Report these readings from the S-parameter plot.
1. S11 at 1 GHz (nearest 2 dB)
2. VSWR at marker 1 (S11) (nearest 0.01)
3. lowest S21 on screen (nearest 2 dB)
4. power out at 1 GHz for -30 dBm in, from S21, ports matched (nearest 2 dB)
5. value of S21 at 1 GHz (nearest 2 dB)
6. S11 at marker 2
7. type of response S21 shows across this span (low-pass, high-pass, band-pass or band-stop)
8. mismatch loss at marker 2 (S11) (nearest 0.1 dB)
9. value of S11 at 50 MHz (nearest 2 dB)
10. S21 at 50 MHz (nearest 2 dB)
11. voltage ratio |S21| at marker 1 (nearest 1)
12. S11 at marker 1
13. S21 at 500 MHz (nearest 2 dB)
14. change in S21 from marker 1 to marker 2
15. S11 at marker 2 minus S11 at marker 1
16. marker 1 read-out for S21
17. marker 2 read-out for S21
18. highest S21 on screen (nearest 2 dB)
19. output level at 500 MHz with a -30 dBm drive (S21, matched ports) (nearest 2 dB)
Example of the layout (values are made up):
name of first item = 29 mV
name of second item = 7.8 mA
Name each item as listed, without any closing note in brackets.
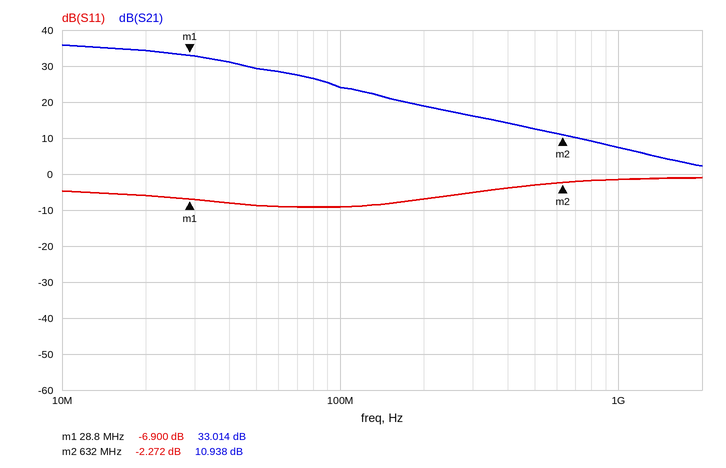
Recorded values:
S11 at 1 GHz = -2 dB
VSWR at marker 1 (S11) = 2.65
lowest S21 on screen = 2 dB
power out at 1 GHz for -30 dBm in, from S21, ports matched = -22 dBm
value of S21 at 1 GHz = 8 dB
S11 at marker 2 = -2.272 dB
type of response S21 shows across this span = low-pass
mismatch loss at marker 2 (S11) = 3.9 dB
value of S11 at 50 MHz = -8 dB
S21 at 50 MHz = 30 dB
voltage ratio |S21| at marker 1 = 45
S11 at marker 1 = -6.900 dB
S21 at 500 MHz = 12 dB
change in S21 from marker 1 to marker 2 = -22.076 dB
S11 at marker 2 minus S11 at marker 1 = 4.628 dB
marker 1 read-out for S21 = 33.014 dB
marker 2 read-out for S21 = 10.938 dB
highest S21 on screen = 36 dB
output level at 500 MHz with a -30 dBm drive (S21, matched ports) = -18 dBm
